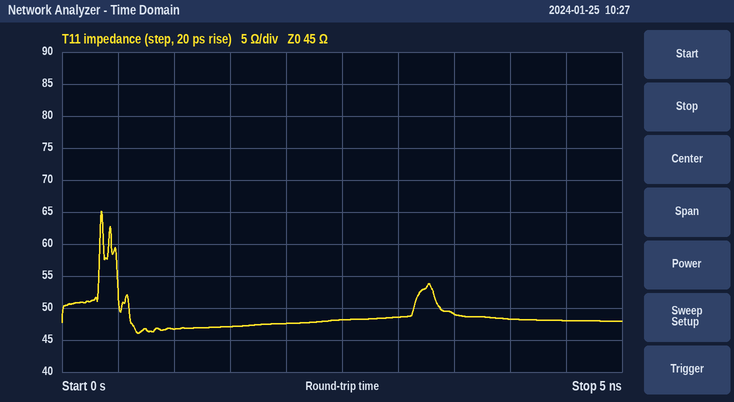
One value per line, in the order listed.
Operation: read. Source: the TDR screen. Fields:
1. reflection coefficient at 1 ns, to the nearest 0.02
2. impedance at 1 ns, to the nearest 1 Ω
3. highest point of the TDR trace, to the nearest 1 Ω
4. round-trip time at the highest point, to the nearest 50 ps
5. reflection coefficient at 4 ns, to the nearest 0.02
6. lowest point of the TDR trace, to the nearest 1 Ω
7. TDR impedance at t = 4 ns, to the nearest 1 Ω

+0.02
47 Ω
65 Ω
350 ps
+0.04
46 Ω
48 Ω
